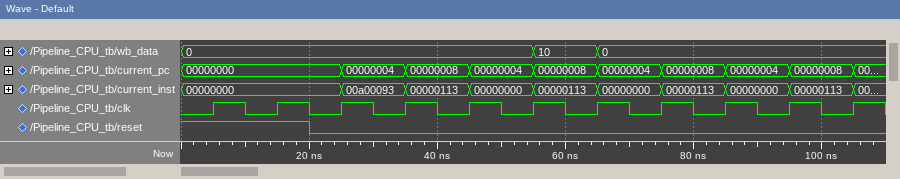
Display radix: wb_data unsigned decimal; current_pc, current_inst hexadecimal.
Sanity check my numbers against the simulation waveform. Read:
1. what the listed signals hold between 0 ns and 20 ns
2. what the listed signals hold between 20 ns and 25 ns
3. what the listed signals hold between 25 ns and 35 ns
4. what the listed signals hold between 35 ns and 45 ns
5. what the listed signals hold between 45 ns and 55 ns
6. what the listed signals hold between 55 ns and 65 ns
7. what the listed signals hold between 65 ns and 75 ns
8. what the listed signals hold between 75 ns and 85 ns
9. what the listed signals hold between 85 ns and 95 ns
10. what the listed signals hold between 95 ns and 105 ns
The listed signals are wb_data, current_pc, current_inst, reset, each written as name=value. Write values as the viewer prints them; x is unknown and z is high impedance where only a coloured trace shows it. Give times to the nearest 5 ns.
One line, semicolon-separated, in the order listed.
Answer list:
wb_data=0, current_pc=00000000, current_inst=00000000, reset=1; wb_data=0, current_pc=00000000, current_inst=00000000, reset=0; wb_data=0, current_pc=00000004, current_inst=00a00093, reset=0; wb_data=0, current_pc=00000008, current_inst=00000113, reset=0; wb_data=0, current_pc=00000004, current_inst=00000000, reset=0; wb_data=10, current_pc=00000008, current_inst=00000113, reset=0; wb_data=0, current_pc=00000004, current_inst=00000000, reset=0; wb_data=0, current_pc=00000008, current_inst=00000113, reset=0; wb_data=0, current_pc=00000004, current_inst=00000000, reset=0; wb_data=0, current_pc=00000008, current_inst=00000113, reset=0
